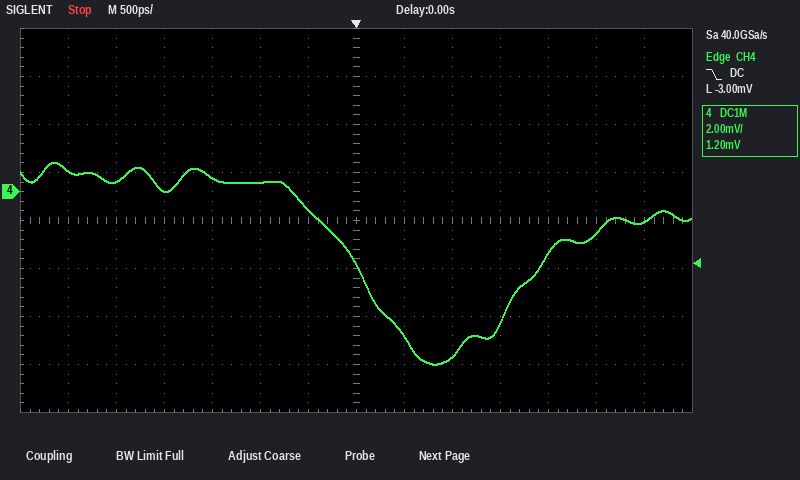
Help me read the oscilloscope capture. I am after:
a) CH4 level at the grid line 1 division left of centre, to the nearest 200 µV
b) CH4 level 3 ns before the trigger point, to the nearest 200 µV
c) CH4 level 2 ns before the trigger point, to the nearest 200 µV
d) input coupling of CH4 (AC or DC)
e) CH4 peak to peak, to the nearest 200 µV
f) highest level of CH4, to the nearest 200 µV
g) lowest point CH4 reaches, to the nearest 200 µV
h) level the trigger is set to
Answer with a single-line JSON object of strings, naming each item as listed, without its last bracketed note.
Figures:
{"CH4 level at the grid line 1 division left of centre, to the nearest 200 µV": "-800 µV", "CH4 level 3 ns before the trigger point, to the nearest 200 µV": "800 µV", "CH4 level 2 ns before the trigger point, to the nearest 200 µV": "0.0 mV", "input coupling of CH4": "DC", "CH4 peak to peak, to the nearest 200 µV": "8.4 mV", "highest level of CH4, to the nearest 200 µV": "1.2 mV", "lowest point CH4 reaches, to the nearest 200 µV": "-7.2 mV", "level the trigger is set to": "-3.00 mV"}
